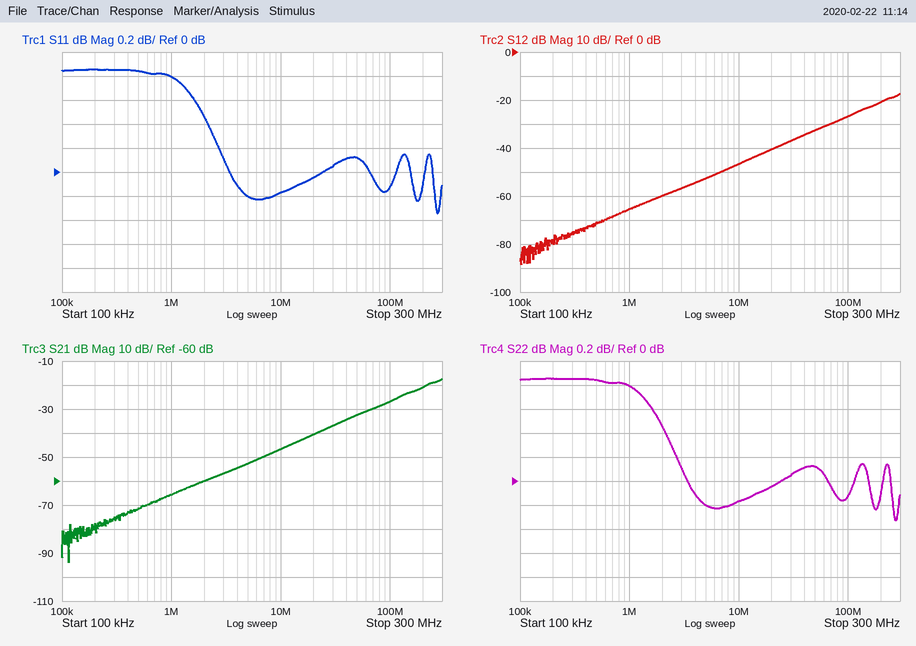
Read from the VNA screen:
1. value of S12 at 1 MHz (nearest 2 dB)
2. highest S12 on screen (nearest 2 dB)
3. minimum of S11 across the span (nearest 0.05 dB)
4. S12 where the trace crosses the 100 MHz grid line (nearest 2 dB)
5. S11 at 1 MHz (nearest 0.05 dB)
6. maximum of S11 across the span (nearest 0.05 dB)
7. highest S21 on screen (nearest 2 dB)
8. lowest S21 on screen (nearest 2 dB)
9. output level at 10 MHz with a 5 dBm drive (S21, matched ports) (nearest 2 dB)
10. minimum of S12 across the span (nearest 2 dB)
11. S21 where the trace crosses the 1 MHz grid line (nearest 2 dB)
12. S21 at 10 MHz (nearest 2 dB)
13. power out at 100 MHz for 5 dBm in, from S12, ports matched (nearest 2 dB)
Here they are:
-66 dB
-18 dB
-0.35 dB
-26 dB
0.80 dB
0.85 dB
-18 dB
-94 dB
-42 dBm
-88 dB
-66 dB
-46 dB
-22 dBm
